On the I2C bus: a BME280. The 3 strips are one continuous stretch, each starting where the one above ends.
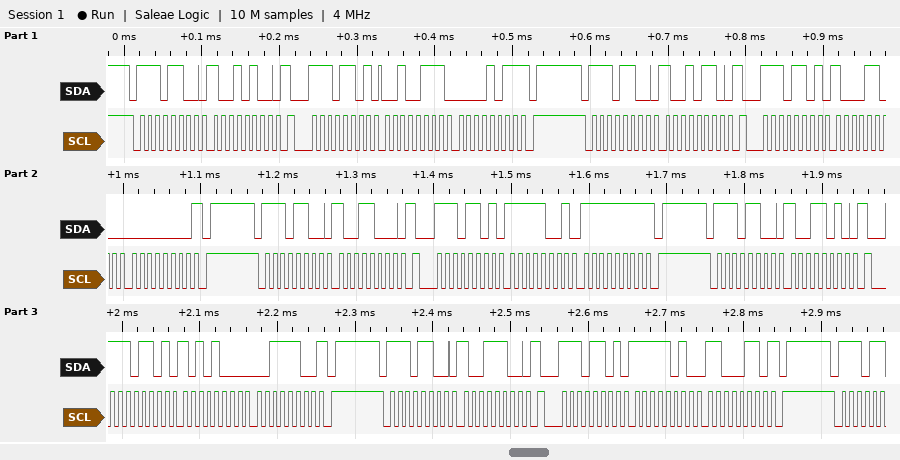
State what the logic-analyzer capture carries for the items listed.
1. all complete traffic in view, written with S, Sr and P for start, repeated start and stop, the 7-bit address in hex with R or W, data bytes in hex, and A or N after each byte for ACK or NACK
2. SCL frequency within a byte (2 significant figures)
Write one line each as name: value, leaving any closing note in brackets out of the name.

all complete traffic in view, written with S, Sr and P for start, repeated start and stop, the 7-bit address in hex with R or W, data bytes in hex, and A or N after each byte for ACK or NACK: S 76W A 94 A Sr 76R A 27 A 0B N P S 76W A 96 A Sr 76R A 8C A 00 N P S 76W A 98 A Sr 76R A F9 A FF N P S 76W A 9A A Sr 76R A A8 A 3C N P S 76W A 9C A Sr 76R A FA A C6 N P
SCL frequency within a byte: 100 kHz
